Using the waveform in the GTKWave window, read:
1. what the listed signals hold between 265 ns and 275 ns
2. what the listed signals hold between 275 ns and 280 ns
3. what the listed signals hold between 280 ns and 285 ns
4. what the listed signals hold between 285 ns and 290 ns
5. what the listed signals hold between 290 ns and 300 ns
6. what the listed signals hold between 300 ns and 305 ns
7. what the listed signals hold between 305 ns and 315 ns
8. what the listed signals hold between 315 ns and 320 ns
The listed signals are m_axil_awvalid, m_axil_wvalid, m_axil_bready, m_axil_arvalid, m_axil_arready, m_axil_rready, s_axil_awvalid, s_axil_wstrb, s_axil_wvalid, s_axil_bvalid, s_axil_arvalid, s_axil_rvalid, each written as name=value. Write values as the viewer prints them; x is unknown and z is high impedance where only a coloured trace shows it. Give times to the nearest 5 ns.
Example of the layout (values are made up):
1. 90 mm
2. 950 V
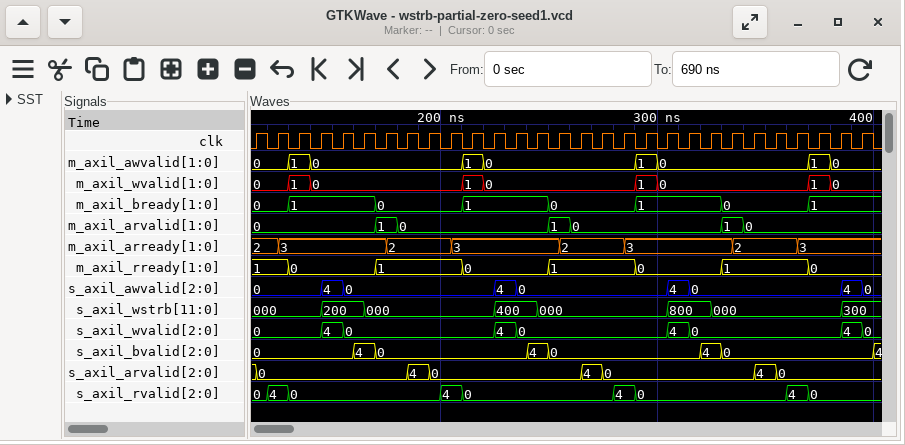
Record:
1. m_axil_awvalid=0, m_axil_wvalid=0, m_axil_bready=0, m_axil_arvalid=0, m_axil_arready=2, m_axil_rready=1, s_axil_awvalid=0, s_axil_wstrb=000, s_axil_wvalid=0, s_axil_bvalid=0, s_axil_arvalid=4, s_axil_rvalid=0
2. m_axil_awvalid=0, m_axil_wvalid=0, m_axil_bready=0, m_axil_arvalid=0, m_axil_arready=2, m_axil_rready=1, s_axil_awvalid=0, s_axil_wstrb=000, s_axil_wvalid=0, s_axil_bvalid=0, s_axil_arvalid=0, s_axil_rvalid=0
3. m_axil_awvalid=0, m_axil_wvalid=0, m_axil_bready=0, m_axil_arvalid=0, m_axil_arready=2, m_axil_rready=1, s_axil_awvalid=0, s_axil_wstrb=000, s_axil_wvalid=0, s_axil_bvalid=0, s_axil_arvalid=0, s_axil_rvalid=4
4. m_axil_awvalid=0, m_axil_wvalid=0, m_axil_bready=0, m_axil_arvalid=0, m_axil_arready=3, m_axil_rready=1, s_axil_awvalid=0, s_axil_wstrb=000, s_axil_wvalid=0, s_axil_bvalid=0, s_axil_arvalid=0, s_axil_rvalid=4
5. m_axil_awvalid=1, m_axil_wvalid=1, m_axil_bready=1, m_axil_arvalid=0, m_axil_arready=3, m_axil_rready=0, s_axil_awvalid=0, s_axil_wstrb=000, s_axil_wvalid=0, s_axil_bvalid=0, s_axil_arvalid=0, s_axil_rvalid=0
6. m_axil_awvalid=0, m_axil_wvalid=0, m_axil_bready=1, m_axil_arvalid=0, m_axil_arready=3, m_axil_rready=0, s_axil_awvalid=0, s_axil_wstrb=000, s_axil_wvalid=0, s_axil_bvalid=0, s_axil_arvalid=0, s_axil_rvalid=0
7. m_axil_awvalid=0, m_axil_wvalid=0, m_axil_bready=1, m_axil_arvalid=0, m_axil_arready=3, m_axil_rready=0, s_axil_awvalid=4, s_axil_wstrb=800, s_axil_wvalid=4, s_axil_bvalid=0, s_axil_arvalid=0, s_axil_rvalid=0
8. m_axil_awvalid=0, m_axil_wvalid=0, m_axil_bready=1, m_axil_arvalid=0, m_axil_arready=3, m_axil_rready=0, s_axil_awvalid=0, s_axil_wstrb=800, s_axil_wvalid=0, s_axil_bvalid=0, s_axil_arvalid=0, s_axil_rvalid=0
